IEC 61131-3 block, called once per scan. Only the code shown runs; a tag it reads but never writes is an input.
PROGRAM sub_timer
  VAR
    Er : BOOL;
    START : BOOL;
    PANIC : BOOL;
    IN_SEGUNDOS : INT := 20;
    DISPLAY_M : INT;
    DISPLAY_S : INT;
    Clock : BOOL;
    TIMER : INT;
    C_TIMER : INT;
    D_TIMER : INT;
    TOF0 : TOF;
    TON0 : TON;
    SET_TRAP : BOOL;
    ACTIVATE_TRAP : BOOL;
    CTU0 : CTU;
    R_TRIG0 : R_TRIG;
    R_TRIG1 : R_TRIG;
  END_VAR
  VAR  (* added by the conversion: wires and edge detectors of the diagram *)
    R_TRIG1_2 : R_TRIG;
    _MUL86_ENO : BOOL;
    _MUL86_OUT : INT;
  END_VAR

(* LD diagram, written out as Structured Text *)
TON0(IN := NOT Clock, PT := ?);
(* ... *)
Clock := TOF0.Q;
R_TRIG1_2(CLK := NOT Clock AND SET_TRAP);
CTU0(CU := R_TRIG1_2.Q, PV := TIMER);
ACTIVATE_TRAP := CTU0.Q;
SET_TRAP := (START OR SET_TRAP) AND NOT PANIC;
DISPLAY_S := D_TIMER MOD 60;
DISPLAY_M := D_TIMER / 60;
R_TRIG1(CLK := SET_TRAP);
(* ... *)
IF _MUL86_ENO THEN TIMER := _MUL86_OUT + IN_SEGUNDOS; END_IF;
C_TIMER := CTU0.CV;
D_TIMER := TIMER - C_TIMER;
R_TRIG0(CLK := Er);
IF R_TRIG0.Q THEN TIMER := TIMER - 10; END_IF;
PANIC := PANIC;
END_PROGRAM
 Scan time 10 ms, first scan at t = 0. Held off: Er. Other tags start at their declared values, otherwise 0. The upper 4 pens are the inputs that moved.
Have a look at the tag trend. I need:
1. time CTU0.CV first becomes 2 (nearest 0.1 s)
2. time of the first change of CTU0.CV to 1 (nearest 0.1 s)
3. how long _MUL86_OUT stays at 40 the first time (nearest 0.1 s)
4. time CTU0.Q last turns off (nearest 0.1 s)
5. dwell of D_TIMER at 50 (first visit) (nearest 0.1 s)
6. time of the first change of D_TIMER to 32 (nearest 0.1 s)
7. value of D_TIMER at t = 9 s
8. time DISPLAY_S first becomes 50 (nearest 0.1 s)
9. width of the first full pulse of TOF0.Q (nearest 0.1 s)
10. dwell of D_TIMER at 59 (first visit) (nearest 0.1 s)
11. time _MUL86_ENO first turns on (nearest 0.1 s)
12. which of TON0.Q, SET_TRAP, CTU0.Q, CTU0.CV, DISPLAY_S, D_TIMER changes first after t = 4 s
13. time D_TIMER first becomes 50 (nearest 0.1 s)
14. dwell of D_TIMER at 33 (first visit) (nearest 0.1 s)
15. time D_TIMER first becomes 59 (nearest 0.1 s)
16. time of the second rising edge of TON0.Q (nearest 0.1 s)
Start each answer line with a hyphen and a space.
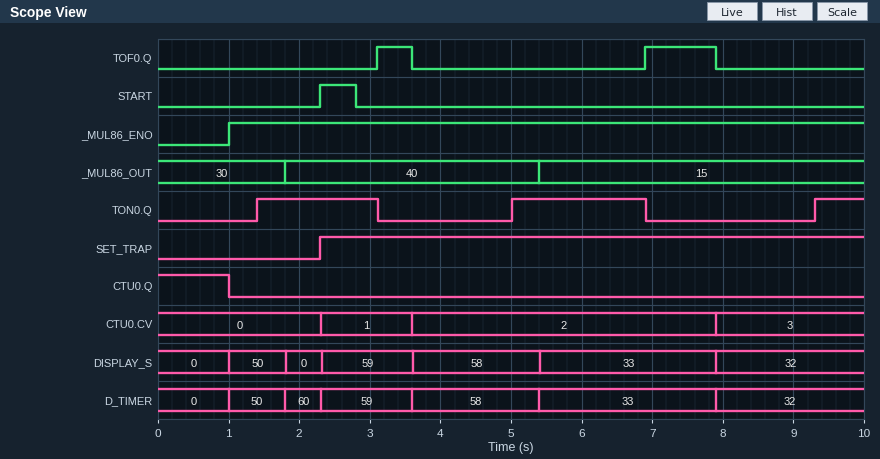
- 3.6 s
- 2.3 s
- 3.6 s
- 1.0 s
- 0.8 s
- 7.9 s
- 32
- 1.0 s
- 0.5 s
- 1.3 s
- 1.0 s
- TON0.Q
- 1.0 s
- 2.5 s
- 2.3 s
- 5.0 s
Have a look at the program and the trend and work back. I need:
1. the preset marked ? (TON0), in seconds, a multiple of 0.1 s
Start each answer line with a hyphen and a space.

- 1.4 s
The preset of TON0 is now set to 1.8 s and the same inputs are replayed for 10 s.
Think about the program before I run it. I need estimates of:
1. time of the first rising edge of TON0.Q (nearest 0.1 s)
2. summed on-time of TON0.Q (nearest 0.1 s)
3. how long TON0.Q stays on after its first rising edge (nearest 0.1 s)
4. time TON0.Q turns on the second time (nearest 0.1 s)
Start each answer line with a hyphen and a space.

- 1.8 s
- 3.1 s
- 1.3 s
- 5.4 s
